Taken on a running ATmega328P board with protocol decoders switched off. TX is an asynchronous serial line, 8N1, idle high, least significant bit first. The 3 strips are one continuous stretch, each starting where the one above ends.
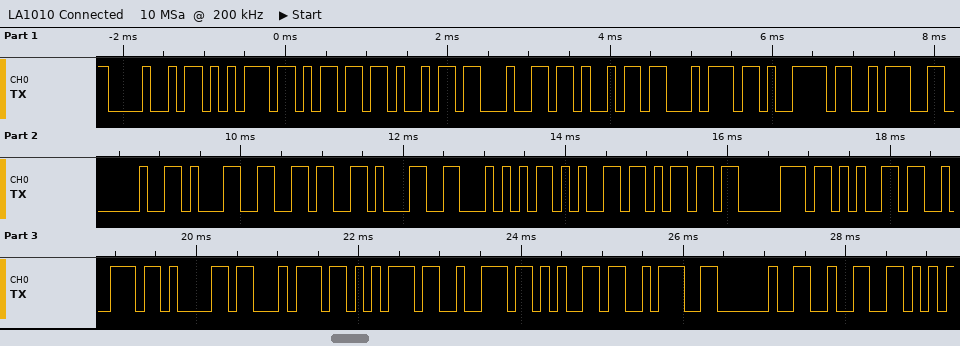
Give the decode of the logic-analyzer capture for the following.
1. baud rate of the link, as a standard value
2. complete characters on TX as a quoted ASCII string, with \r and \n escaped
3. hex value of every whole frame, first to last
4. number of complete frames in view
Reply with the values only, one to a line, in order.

9600 baud
"Humidity: 161Temperature: 2"
48 75 6D 69 64 69 74 79 3A 20 31 36 31 54 65 6D 70 65 72 61 74 75 72 65 3A 20 32
27
